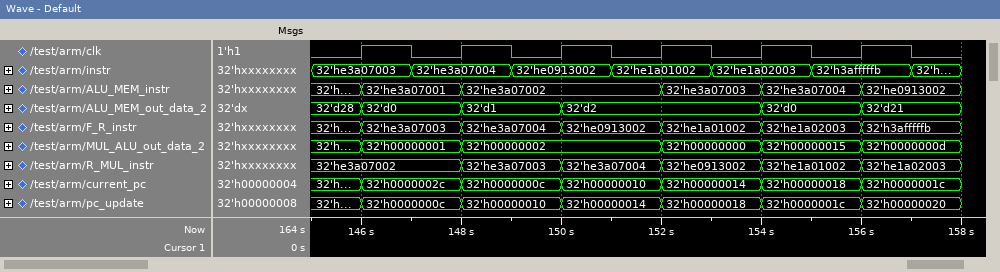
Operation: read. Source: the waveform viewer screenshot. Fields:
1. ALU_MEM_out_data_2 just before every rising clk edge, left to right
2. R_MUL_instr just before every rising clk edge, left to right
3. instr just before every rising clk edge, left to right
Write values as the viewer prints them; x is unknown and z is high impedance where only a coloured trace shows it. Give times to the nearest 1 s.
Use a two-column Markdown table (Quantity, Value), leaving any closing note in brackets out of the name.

| Quantity | Value |
|---|---|
| ALU_MEM_out_data_2 just before every rising clk edge, left to right | 32'd28, 32'd0, 32'd1, 32'd2, 32'd2, 32'd0 |
| R_MUL_instr just before every rising clk edge, left to right | 32'he3a07002, 32'he3a07002, 32'he3a07003, 32'he3a07004, 32'he0913002, 32'he1a01002 |
| instr just before every rising clk edge, left to right | 32'he3a07003, 32'he3a07004, 32'he0913002, 32'he1a01002, 32'he1a02003, 32'h3afffffb |
